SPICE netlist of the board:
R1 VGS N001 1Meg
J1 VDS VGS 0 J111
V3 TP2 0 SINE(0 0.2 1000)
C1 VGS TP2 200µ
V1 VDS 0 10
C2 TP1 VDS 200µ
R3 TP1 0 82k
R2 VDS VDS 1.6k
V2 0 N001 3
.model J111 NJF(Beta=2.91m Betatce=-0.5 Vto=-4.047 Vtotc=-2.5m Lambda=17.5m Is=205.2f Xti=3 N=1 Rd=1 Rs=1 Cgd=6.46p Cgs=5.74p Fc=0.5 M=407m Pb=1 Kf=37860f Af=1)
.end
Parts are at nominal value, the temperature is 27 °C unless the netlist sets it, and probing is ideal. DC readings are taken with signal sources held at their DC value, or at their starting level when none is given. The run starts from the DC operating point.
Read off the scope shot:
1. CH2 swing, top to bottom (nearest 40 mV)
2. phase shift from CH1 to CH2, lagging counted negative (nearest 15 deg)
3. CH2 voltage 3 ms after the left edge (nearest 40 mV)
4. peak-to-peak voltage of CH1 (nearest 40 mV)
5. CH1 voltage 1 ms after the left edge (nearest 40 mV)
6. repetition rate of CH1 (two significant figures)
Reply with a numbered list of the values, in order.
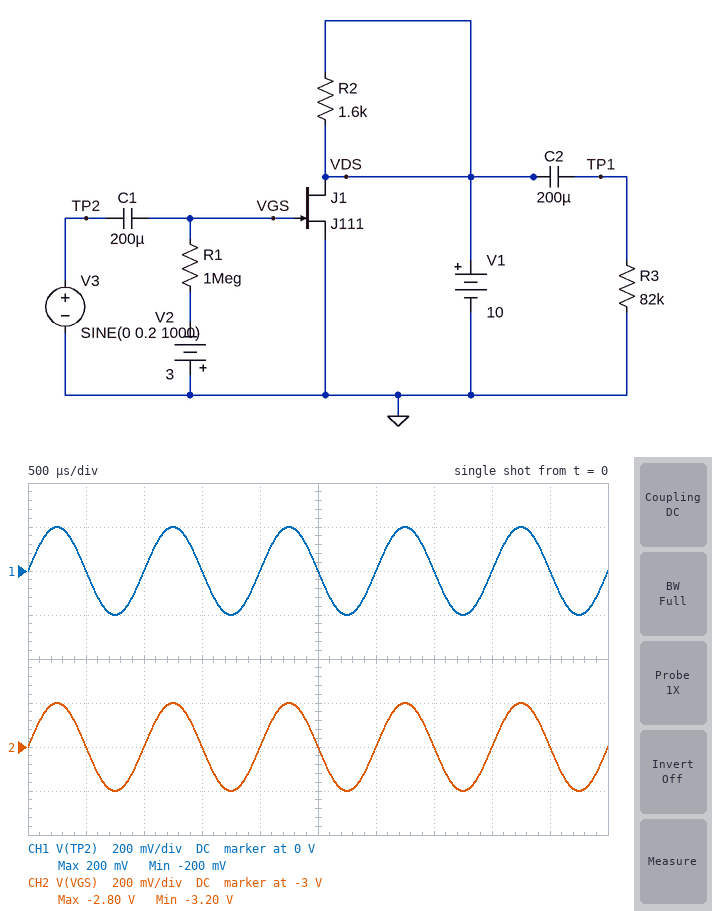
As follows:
1. 400 mV
2. 0 deg
3. -3.00 V
4. 400 mV
5. 0 V
6. 1.0 kHz
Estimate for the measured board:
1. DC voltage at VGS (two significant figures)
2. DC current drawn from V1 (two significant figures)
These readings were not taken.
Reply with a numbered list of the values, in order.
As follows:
1. -3.0 V
2. 3.7 mA
